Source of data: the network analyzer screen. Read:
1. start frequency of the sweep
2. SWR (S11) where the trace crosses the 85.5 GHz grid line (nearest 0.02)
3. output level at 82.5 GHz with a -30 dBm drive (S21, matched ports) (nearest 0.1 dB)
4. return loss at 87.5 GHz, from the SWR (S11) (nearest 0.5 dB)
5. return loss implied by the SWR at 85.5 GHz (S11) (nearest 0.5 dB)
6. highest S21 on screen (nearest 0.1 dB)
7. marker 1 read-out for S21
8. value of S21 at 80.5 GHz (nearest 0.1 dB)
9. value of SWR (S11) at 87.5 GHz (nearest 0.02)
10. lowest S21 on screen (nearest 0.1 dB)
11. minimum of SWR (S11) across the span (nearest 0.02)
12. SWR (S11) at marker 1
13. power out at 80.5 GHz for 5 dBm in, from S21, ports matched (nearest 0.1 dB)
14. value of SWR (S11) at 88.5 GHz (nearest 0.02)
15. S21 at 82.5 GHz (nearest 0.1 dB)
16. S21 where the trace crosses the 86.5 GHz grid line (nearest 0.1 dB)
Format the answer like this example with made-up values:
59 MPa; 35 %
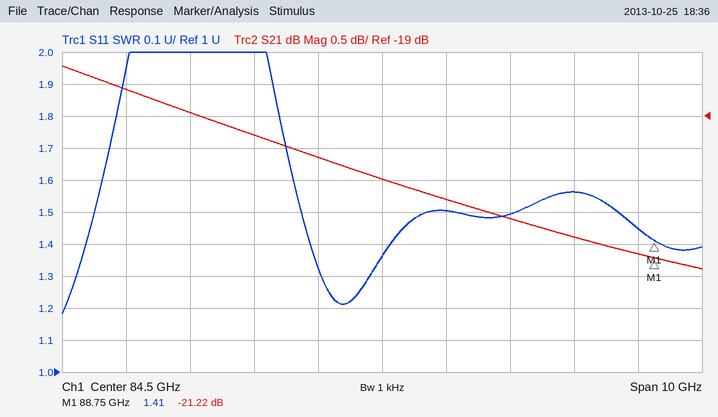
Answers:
79.5 GHz; 1.50; -49.3 dBm; 13.0 dB; 14.0 dB; -18.2 dB; -21.22 dB; -18.6 dB; 1.56; -21.4 dB; 1.18; 1.41; -13.6 dBm; 1.44; -19.3 dB; -20.6 dB
